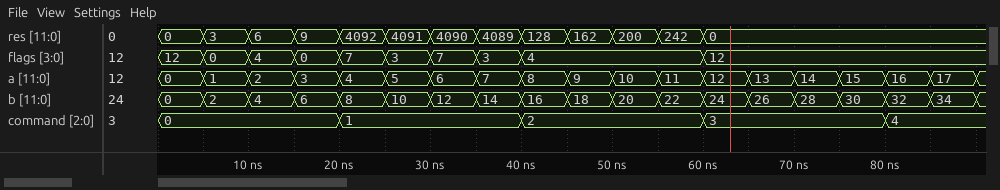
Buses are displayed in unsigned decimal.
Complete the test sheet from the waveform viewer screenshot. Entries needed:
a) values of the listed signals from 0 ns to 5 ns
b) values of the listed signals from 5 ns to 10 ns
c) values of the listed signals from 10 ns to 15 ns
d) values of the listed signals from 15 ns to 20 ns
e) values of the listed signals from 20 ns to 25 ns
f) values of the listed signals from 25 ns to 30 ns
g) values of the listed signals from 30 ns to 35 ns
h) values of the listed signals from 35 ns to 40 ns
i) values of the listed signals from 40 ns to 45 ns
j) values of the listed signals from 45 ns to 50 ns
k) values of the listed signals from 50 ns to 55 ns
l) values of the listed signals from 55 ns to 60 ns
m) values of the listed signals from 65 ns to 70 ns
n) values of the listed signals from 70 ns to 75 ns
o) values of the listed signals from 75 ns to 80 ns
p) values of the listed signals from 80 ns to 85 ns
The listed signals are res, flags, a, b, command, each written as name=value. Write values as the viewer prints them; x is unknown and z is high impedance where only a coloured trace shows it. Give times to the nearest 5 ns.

res=0, flags=12, a=0, b=0, command=0
res=3, flags=0, a=1, b=2, command=0
res=6, flags=4, a=2, b=4, command=0
res=9, flags=0, a=3, b=6, command=0
res=4092, flags=7, a=4, b=8, command=1
res=4091, flags=3, a=5, b=10, command=1
res=4090, flags=7, a=6, b=12, command=1
res=4089, flags=3, a=7, b=14, command=1
res=128, flags=4, a=8, b=16, command=2
res=162, flags=4, a=9, b=18, command=2
res=200, flags=4, a=10, b=20, command=2
res=242, flags=4, a=11, b=22, command=2
res=0, flags=12, a=13, b=26, command=3
res=0, flags=12, a=14, b=28, command=3
res=0, flags=12, a=15, b=30, command=3
res=0, flags=12, a=16, b=32, command=4
